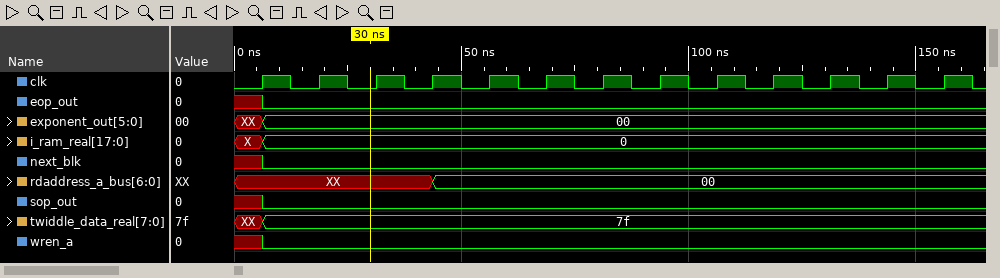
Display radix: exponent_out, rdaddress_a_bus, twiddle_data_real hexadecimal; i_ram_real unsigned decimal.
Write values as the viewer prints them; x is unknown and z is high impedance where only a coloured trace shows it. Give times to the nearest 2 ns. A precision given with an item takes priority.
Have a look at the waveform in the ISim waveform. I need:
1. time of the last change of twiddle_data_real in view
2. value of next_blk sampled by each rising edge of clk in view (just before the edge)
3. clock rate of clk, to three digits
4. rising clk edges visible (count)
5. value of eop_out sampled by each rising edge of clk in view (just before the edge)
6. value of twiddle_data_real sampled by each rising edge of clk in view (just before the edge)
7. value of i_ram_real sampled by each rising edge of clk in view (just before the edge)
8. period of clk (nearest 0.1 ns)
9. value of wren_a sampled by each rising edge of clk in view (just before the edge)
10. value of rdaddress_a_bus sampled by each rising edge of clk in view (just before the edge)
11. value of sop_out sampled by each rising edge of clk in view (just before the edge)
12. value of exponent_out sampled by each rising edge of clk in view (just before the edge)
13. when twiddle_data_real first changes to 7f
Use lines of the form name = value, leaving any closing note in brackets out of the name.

time of the last change of twiddle_data_real in view = 6 ns
value of next_blk sampled by each rising edge of clk in view = x 0 0 0 0 0 0 0 0 0 0 0 0
clock rate of clk, to three digits = 80.0 MHz
rising clk edges visible = 13
value of eop_out sampled by each rising edge of clk in view = x 0 0 0 0 0 0 0 0 0 0 0 0
value of twiddle_data_real sampled by each rising edge of clk in view = XX, 7f, 7f, 7f, 7f, 7f, 7f, 7f, 7f, 7f, 7f, 7f, 7f
value of i_ram_real sampled by each rising edge of clk in view = X, 0, 0, 0, 0, 0, 0, 0, 0, 0, 0, 0, 0
period of clk = 12.5 ns
value of wren_a sampled by each rising edge of clk in view = x 0 0 0 0 0 0 0 0 0 0 0 0
value of rdaddress_a_bus sampled by each rising edge of clk in view = XX, XX, XX, XX, 00, 00, 00, 00, 00, 00, 00, 00, 00
value of sop_out sampled by each rising edge of clk in view = x 0 0 0 0 0 0 0 0 0 0 0 0
value of exponent_out sampled by each rising edge of clk in view = XX, 00, 00, 00, 00, 00, 00, 00, 00, 00, 00, 00, 00
when twiddle_data_real first changes to 7f = 6 ns
